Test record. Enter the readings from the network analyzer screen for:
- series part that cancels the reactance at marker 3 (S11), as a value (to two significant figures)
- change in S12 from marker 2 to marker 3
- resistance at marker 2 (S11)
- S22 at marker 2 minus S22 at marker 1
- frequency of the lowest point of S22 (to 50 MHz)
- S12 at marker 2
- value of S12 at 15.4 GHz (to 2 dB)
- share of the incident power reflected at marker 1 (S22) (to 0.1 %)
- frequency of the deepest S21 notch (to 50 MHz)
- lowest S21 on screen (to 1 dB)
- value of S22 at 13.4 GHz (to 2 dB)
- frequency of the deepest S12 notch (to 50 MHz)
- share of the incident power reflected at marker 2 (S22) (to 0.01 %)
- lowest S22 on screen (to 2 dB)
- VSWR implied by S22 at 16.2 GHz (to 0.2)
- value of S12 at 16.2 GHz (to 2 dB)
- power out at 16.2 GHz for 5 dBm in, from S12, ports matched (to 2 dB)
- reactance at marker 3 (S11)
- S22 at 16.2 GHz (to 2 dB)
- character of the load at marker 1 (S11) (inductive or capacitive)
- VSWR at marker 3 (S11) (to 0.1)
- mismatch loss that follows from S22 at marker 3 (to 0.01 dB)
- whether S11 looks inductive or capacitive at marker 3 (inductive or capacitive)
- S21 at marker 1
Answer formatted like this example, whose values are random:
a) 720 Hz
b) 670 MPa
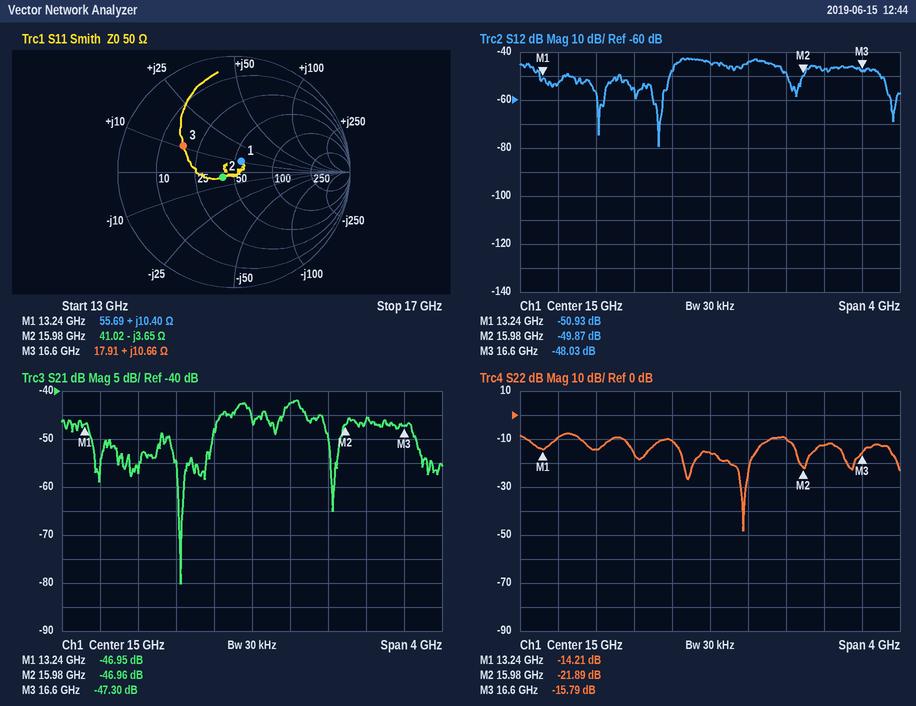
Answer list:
a) 900 fF
b) 1.84 dB
c) 41.02 Ω
d) -7.68 dB
e) 15.35 GHz
f) -49.87 dB
g) -44 dB
h) 3.8 %
i) 14.25 GHz
j) -80 dB
k) -10 dB
l) 14.45 GHz
m) 0.65 %
n) -48 dB
o) 1.6
p) -48 dB
q) -42 dBm
r) +10.66 Ω
s) -12 dB
t) inductive
u) 2.9
v) 0.12 dB
w) inductive
x) -46.95 dB
